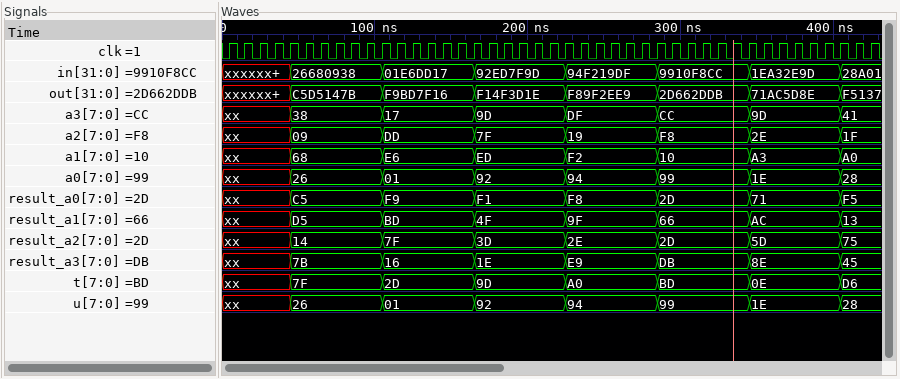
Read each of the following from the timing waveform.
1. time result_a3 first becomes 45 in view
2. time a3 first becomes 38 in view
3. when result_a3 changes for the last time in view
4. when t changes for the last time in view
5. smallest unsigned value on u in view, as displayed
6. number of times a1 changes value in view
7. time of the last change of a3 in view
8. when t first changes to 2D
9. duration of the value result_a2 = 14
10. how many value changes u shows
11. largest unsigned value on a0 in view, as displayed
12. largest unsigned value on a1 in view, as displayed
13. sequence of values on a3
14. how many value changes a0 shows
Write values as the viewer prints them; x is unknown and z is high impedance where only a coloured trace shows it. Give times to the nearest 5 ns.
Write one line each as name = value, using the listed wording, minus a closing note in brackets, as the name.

time result_a3 first becomes 45 in view = 405 ns
time a3 first becomes 38 in view = 45 ns
when result_a3 changes for the last time in view = 405 ns
when t changes for the last time in view = 405 ns
smallest unsigned value on u in view, as displayed = 01
number of times a1 changes value in view = 7
time of the last change of a3 in view = 405 ns
when t first changes to 2D = 105 ns
duration of the value result_a2 = 14 = 60 ns
how many value changes u shows = 7
largest unsigned value on a0 in view, as displayed = 99
largest unsigned value on a1 in view, as displayed = F2
sequence of values on a3 = xx, 38, 17, 9D, DF, CC, 9D, 41
how many value changes a0 shows = 7
